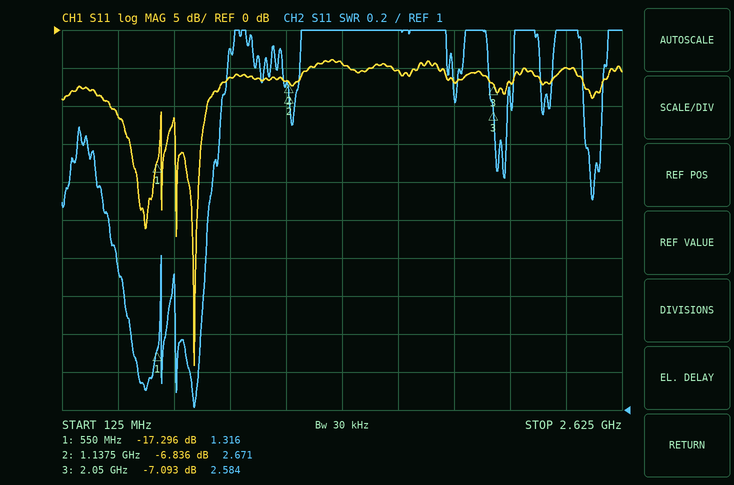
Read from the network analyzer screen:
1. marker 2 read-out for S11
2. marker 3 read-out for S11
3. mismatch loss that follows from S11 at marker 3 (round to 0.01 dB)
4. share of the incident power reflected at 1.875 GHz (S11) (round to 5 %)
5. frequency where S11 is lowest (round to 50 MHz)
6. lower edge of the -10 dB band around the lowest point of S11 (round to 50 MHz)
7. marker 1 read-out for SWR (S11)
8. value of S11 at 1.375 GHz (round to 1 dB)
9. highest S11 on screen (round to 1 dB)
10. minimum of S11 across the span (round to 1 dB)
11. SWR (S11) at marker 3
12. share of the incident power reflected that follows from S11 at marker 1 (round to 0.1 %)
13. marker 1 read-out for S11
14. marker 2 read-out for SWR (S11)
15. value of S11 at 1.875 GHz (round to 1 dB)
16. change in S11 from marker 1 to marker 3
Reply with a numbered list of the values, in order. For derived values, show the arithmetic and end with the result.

1. -6.836 dB
2. -7.093 dB
3. −10 log10(1 − 10^(-7.093/10)) ≈ 0.94 dB
4. 10^(-7/10) ≈ 20 %
5. 700 MHz
6. 350 MHz
7. 1.316
8. -4 dB
9. -4 dB
10. -44 dB
11. 2.584
12. 10^(-17.296/10) ≈ 1.9 %
13. -17.296 dB
14. 2.671
15. -7 dB
16. -7.093 − (-17.296) = 10.203 dB
